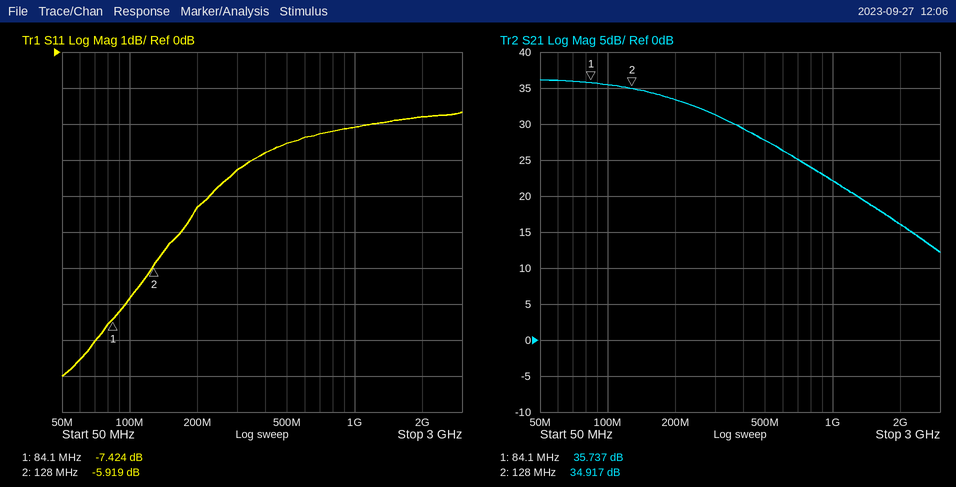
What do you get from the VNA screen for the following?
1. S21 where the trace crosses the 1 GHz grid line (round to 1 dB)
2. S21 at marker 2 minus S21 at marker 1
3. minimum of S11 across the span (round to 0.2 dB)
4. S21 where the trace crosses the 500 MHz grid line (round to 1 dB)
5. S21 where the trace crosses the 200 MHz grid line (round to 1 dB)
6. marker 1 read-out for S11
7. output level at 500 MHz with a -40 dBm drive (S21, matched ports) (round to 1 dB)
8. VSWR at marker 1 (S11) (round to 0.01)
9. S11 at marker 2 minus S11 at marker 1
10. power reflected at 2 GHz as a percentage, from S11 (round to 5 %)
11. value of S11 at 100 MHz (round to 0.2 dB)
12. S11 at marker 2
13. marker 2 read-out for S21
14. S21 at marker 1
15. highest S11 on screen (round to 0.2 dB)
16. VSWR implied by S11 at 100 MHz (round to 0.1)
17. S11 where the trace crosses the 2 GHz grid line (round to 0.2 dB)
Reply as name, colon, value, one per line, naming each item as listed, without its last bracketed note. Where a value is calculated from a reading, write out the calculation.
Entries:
S21 where the trace crosses the 1 GHz grid line: 22 dB
S21 at marker 2 minus S21 at marker 1: 34.917 − (35.737) = -0.820 dB
minimum of S11 across the span: -9.0 dB
S21 where the trace crosses the 500 MHz grid line: 28 dB
S21 where the trace crosses the 200 MHz grid line: 33 dB
marker 1 read-out for S11: -7.424 dB
output level at 500 MHz with a -40 dBm drive (S21, matched ports): -40 dBm + (28 dB) = -12 dBm
VSWR at marker 1 (S11): (1 + 0.4254)/(1 − 0.4254) ≈ 2.48
S11 at marker 2 minus S11 at marker 1: -5.919 − (-7.424) = 1.505 dB
power reflected at 2 GHz as a percentage, from S11: 10^(-1.8/10) ≈ 66.1 %, so 65 % to the nearest 5 %
value of S11 at 100 MHz: -6.8 dB
S11 at marker 2: -5.919 dB
marker 2 read-out for S21: 34.917 dB
S21 at marker 1: 35.737 dB
highest S11 on screen: -1.6 dB
VSWR implied by S11 at 100 MHz: |Γ| = 10^(-6.8/20) = 0.4571; VSWR = (1 + 0.4571)/(1 − 0.4571) ≈ 2.7
S11 where the trace crosses the 2 GHz grid line: -1.8 dB
